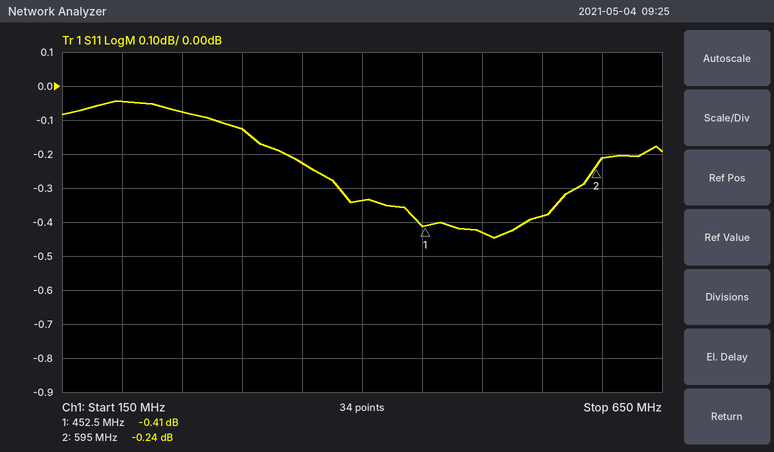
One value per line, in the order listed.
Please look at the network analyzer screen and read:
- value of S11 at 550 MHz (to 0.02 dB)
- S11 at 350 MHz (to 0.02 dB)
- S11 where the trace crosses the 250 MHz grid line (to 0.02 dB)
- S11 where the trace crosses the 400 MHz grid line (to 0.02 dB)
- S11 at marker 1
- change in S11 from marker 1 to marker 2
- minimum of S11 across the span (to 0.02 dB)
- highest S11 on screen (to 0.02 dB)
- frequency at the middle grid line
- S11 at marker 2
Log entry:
-0.38 dB
-0.22 dB
-0.08 dB
-0.34 dB
-0.41 dB
0.17 dB
-0.44 dB
-0.04 dB
400 MHz
-0.24 dB
